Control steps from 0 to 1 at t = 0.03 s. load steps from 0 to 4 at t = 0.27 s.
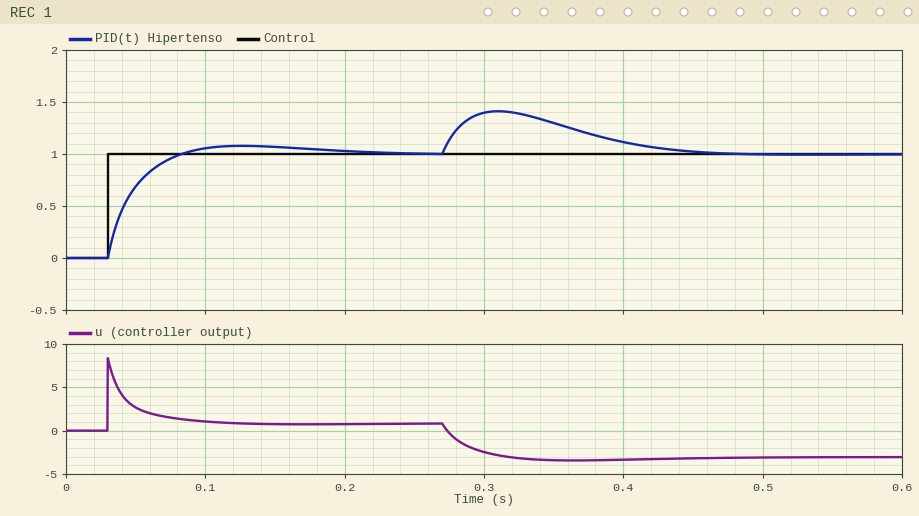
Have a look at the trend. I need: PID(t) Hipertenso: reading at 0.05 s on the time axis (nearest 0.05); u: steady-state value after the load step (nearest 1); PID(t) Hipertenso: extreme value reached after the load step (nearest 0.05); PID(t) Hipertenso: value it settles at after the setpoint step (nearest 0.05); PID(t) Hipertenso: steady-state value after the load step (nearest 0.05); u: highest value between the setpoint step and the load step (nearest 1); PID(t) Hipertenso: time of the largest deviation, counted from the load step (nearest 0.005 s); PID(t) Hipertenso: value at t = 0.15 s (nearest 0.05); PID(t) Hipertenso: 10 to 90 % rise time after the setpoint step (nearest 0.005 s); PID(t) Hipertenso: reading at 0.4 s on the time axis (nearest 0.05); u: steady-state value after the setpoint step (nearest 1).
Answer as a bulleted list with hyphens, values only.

- 0.70
- -3
- 1.40
- 1.00
- 1.00
- 8
- 0.040 s
- 1.05
- 0.035 s
- 1.10
- 1
